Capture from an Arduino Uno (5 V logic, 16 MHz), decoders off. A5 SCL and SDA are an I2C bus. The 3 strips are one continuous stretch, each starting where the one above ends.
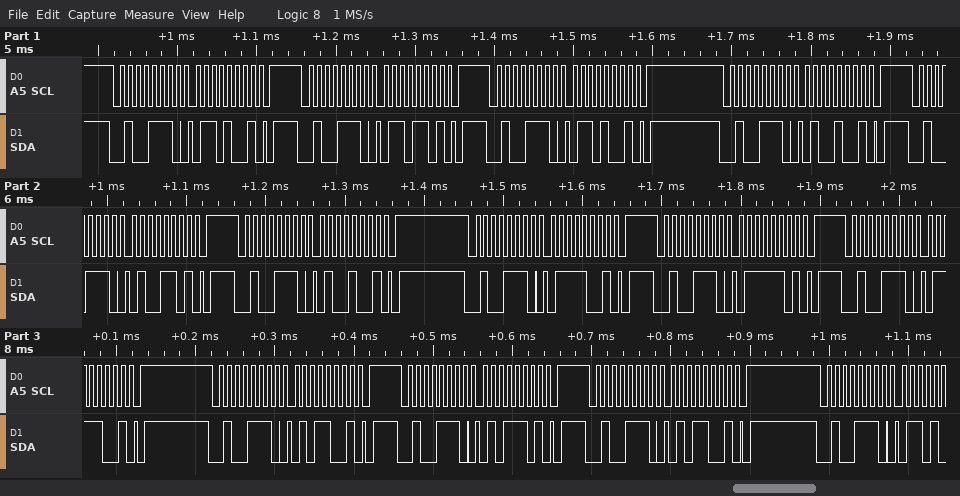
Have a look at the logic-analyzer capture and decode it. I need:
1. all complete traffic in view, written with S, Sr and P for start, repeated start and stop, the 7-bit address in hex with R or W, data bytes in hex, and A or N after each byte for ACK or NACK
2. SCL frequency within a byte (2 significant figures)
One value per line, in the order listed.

S 27W A 69 A P S 27W A 6D A P S 27W A 69 A P S 27W A 49 A P S 27W A 4D A P S 27W A 49 A P S 27W A 79 A P S 27W A 7D A P S 27W A 79 A P S 27W A 59 A P S 27W A 5D A P S 27W A 59 A P S 27W A
100 kHz
